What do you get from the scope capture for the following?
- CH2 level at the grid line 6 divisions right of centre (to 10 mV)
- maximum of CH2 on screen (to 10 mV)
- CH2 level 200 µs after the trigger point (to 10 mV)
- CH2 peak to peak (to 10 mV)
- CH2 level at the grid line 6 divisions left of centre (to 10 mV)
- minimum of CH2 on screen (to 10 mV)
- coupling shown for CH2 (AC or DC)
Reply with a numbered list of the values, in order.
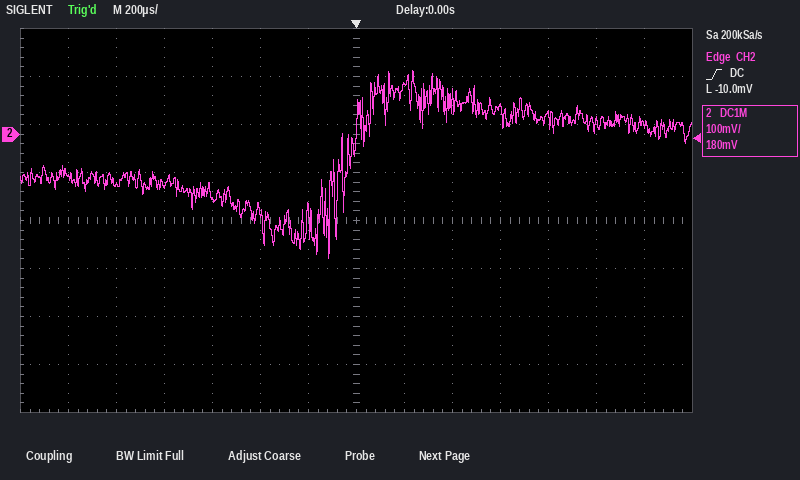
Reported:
1. 20 mV
2. 130 mV
3. 100 mV
4. 390 mV
5. -90 mV
6. -260 mV
7. DC
